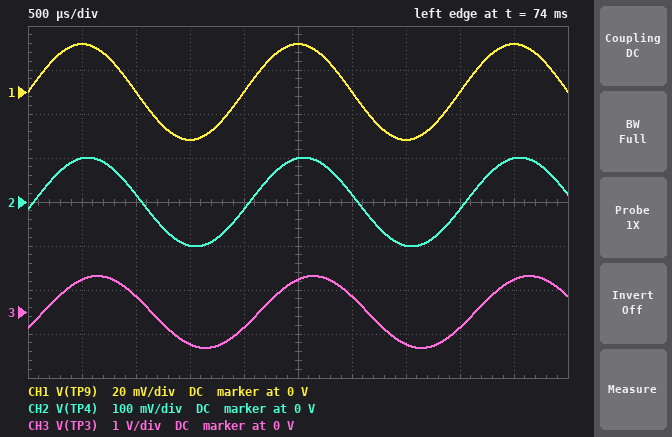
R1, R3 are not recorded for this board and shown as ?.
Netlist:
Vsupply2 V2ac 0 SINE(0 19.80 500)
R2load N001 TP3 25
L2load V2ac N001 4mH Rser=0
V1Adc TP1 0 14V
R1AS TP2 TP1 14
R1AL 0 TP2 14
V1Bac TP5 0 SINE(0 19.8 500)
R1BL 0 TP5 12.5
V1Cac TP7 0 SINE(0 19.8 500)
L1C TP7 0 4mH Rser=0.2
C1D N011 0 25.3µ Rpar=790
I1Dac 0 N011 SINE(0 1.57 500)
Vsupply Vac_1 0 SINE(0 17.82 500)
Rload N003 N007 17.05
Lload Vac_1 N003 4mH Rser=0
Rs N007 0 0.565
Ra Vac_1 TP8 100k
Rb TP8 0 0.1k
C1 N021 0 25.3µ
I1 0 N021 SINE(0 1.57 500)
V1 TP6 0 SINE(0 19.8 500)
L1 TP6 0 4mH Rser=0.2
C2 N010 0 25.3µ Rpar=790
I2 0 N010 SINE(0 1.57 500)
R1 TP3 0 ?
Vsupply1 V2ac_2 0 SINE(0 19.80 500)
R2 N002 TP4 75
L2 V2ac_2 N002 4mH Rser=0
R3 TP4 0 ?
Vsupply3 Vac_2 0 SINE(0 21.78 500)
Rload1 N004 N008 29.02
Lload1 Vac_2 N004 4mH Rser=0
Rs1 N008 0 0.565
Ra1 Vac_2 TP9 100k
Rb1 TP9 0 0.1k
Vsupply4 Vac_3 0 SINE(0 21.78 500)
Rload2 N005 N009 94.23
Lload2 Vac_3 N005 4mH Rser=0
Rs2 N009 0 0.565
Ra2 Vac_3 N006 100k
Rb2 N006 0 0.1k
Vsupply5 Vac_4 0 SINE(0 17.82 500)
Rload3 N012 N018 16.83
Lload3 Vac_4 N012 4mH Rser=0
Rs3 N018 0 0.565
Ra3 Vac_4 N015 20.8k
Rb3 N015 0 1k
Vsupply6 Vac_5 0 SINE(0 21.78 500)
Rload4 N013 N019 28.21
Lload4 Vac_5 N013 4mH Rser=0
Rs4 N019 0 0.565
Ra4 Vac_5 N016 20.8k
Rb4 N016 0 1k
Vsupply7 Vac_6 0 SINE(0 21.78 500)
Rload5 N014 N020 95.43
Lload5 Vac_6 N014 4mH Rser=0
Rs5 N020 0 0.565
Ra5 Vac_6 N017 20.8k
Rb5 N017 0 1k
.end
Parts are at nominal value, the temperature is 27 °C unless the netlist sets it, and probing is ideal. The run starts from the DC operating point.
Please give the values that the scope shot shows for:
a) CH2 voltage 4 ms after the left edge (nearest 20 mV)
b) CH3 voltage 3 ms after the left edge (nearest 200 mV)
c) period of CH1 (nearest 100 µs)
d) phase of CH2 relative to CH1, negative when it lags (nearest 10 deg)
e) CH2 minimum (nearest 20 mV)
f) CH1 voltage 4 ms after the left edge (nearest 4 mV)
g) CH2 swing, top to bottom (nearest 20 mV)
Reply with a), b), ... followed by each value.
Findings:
a) -20 mV
b) 400 mV
c) 2.0 ms
d) -10 deg
e) -100 mV
f) 0 V
g) 200 mV
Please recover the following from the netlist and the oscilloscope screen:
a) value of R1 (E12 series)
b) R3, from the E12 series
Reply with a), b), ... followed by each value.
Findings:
a) 1.2 Ω
b) 0.39 Ω
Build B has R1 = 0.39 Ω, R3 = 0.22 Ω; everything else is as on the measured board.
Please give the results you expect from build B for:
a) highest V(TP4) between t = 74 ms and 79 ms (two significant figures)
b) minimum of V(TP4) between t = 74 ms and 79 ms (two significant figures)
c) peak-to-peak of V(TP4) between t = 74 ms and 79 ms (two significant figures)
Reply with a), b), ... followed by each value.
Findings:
a) 57 mV
b) -57 mV
c) 110 mV
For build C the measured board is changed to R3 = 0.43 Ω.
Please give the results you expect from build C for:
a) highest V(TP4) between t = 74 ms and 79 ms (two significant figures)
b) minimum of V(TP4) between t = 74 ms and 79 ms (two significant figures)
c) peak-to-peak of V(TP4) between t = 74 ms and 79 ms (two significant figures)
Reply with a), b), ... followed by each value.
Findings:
a) 110 mV
b) -110 mV
c) 220 mV
